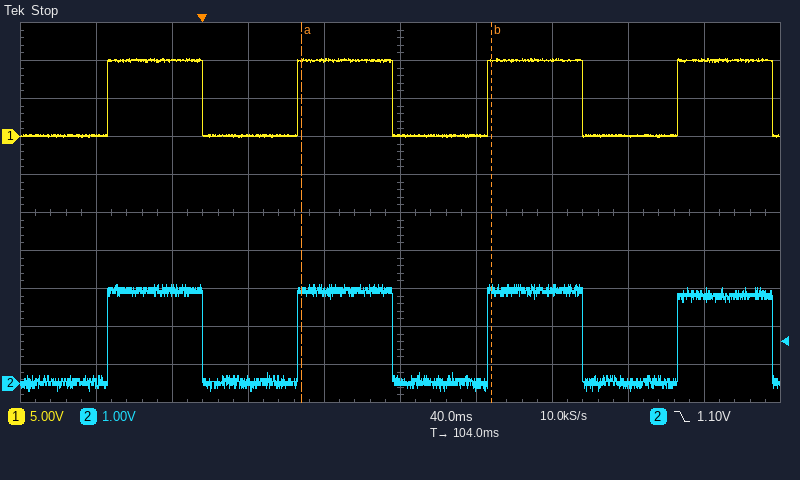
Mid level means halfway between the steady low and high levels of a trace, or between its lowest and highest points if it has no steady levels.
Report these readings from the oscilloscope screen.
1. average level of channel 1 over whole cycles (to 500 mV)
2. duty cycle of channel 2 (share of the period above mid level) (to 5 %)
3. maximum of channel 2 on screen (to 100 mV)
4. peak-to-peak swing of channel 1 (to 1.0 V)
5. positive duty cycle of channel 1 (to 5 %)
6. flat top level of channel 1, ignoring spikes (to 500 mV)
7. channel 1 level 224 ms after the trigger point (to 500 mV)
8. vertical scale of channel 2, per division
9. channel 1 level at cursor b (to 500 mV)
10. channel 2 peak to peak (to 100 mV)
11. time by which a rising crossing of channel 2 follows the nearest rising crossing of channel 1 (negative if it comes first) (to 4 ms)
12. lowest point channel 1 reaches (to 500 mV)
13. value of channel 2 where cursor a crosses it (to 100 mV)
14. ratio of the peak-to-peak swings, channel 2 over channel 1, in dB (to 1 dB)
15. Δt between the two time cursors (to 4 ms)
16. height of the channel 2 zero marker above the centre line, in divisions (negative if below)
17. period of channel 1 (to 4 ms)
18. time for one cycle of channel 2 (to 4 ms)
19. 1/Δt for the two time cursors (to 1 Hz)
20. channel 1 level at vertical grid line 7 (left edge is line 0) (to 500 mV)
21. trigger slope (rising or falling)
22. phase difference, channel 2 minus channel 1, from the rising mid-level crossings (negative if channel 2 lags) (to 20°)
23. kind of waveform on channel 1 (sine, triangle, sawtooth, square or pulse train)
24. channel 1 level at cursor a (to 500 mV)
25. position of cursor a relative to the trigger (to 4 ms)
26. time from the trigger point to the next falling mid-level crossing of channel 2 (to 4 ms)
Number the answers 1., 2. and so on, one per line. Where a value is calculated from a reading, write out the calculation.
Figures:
1. 0.0 V + 0.5 × (10.0 V − (0.0 V)) ≈ 5.0 V
2. 50 %
3. 2.6 V
4. 10.0 V
5. 50 %
6. 10.0 V
7. 0.0 V
8. 1 V
9. 10.0 V
10. 2.6 V − (-200 mV) = 2.8 V
11. 0 ms
12. 0.0 V
13. 2.4 V
14. 20 log10(2.8 V / 10.0 V) ≈ -11 dB
15. 100 ms
16. -4.5 div
17. 100 ms
18. 100 ms
19. 1 / 100 ms ≈ 10 Hz
20. 10.0 V
21. falling
22. −360° × (0 ms) / 100 ms ≈ 0°
23. square
24. 10.0 V
25. +52 ms
26. 100 ms
